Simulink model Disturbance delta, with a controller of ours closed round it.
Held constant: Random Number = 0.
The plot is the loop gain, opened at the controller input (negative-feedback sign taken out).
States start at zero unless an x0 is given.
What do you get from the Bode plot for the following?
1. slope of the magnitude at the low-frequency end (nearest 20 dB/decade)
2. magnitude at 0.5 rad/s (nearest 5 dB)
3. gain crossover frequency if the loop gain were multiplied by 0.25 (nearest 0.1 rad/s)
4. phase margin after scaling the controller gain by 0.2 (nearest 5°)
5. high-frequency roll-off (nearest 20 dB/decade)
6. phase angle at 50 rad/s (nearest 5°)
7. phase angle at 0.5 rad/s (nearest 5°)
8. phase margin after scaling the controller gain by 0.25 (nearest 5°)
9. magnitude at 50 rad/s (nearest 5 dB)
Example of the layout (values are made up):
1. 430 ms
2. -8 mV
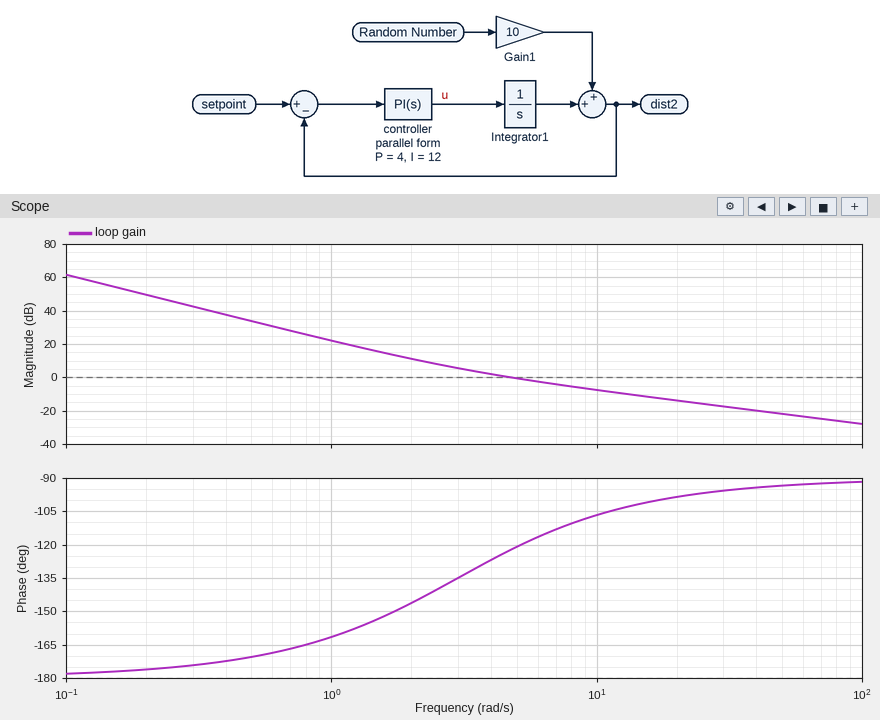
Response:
1. -40 dB/decade
2. 35 dB
3. 1.9 rad/s
4. 30°
5. -20 dB/decade
6. -95°
7. -170°
8. 30°
9. -20 dB
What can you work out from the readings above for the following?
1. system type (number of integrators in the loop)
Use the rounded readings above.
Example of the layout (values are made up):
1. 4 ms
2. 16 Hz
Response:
1. 2
